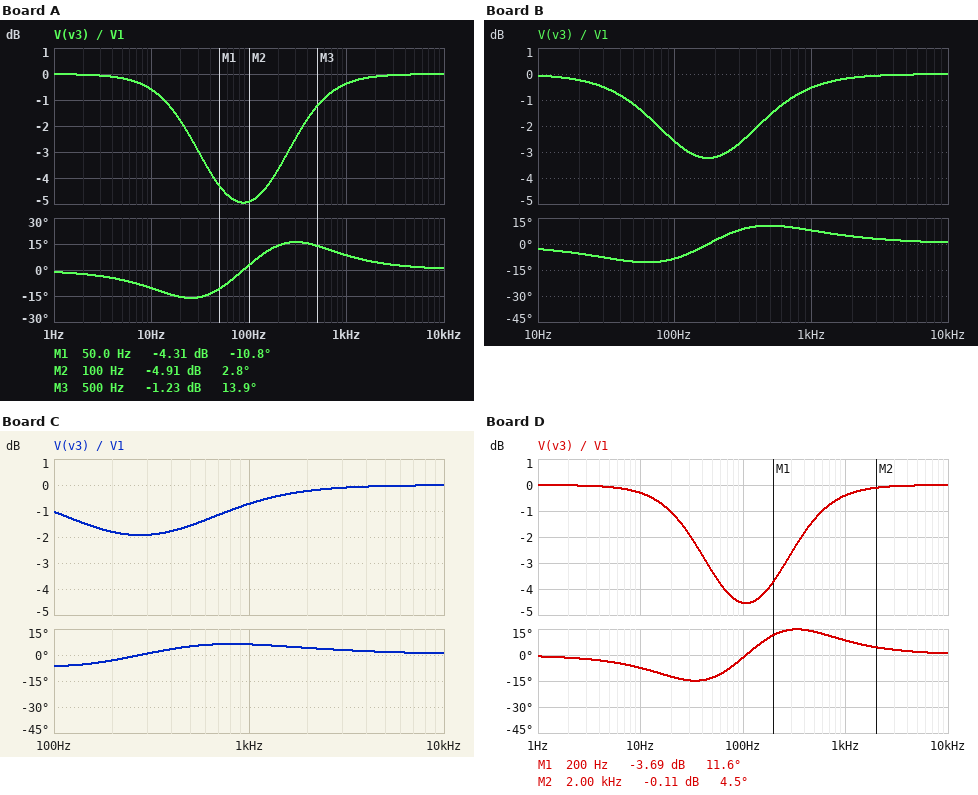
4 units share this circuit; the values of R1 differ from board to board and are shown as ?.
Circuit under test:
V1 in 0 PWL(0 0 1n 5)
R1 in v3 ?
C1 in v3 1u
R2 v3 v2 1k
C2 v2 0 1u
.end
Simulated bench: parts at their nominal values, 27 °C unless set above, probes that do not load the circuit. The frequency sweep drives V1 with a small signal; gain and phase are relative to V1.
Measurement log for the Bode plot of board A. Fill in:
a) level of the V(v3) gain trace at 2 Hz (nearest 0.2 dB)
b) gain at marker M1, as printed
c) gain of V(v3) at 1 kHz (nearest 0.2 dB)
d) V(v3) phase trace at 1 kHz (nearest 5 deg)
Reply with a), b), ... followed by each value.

a) 0 dB
b) -4.31 dB
c) -0.4 dB
d) 10 deg
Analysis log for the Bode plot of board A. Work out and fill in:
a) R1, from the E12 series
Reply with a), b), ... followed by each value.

a) 3.3 kΩ
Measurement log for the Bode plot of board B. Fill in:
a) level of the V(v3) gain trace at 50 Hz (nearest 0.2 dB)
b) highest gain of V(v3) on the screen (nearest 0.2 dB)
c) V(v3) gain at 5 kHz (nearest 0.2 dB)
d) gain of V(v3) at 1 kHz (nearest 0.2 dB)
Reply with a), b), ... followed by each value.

a) -1.2 dB
b) 0 dB
c) 0 dB
d) -0.6 dB
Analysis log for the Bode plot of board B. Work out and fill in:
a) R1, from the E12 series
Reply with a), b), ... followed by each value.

a) 820 Ω
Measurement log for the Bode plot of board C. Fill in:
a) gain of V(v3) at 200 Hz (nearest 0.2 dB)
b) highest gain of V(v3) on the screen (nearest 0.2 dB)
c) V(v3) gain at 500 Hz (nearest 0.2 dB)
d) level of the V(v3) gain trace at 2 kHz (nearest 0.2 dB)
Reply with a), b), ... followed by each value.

a) -1.8 dB
b) 0 dB
c) -1.6 dB
d) -0.2 dB
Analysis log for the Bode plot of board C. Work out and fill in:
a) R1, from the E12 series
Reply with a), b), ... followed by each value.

a) 330 Ω
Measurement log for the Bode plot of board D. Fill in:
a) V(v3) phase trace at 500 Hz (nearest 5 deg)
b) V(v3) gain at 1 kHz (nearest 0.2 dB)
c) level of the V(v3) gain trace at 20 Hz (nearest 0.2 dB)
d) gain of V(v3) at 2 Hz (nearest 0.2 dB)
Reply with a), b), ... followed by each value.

a) 15 deg
b) -0.4 dB
c) -1.0 dB
d) 0 dB
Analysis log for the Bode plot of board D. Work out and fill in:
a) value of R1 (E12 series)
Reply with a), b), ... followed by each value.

a) 2.2 kΩ
